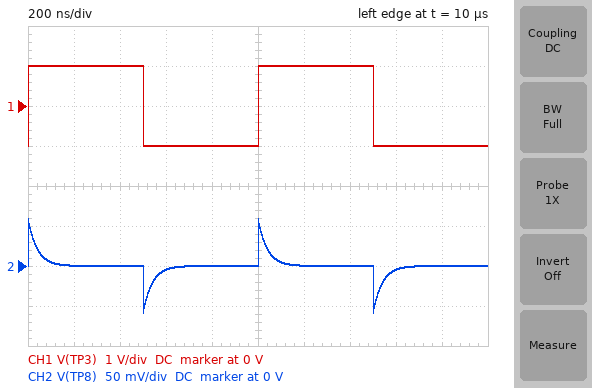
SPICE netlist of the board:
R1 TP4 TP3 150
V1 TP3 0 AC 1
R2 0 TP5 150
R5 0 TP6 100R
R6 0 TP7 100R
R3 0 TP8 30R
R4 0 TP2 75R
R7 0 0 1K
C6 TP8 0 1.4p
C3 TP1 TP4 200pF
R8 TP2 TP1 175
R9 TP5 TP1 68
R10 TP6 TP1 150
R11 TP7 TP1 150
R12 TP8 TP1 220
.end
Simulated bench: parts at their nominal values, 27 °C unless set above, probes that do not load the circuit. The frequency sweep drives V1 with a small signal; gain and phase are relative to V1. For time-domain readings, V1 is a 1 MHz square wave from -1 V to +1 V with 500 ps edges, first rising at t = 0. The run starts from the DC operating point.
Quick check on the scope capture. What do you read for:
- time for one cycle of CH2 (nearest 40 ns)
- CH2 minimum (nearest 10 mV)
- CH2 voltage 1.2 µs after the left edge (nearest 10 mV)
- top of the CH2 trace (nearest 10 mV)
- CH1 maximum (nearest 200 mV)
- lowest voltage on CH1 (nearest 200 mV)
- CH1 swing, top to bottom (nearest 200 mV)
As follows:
1.00 µs
-60 mV
0 V
60 mV
1.0 V
-1.0 V
2.0 V
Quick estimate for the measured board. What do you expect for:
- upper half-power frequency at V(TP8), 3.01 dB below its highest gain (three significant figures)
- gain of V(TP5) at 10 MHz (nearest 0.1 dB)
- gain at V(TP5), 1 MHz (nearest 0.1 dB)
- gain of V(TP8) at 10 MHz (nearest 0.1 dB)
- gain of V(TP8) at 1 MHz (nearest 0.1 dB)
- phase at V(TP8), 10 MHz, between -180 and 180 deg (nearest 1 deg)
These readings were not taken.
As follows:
4.23 GHz
-16.1 dB
-27.8 dB
-31.3 dB
-43.0 dB
22 deg
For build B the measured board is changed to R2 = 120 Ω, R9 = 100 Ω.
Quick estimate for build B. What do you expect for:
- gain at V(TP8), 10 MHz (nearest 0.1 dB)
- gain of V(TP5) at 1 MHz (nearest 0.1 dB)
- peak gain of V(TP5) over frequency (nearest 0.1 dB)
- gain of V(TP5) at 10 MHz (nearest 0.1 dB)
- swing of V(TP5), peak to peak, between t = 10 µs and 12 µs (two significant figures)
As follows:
-31.3 dB
-29.8 dB
-17.5 dB
-18.1 dB
530 mV
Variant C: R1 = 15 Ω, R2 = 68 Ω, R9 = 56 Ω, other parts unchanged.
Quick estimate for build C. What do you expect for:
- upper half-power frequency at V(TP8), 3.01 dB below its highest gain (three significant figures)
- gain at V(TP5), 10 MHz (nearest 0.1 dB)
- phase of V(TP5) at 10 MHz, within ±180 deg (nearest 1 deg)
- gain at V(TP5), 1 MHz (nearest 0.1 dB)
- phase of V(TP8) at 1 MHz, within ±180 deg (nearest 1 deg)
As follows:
4.31 GHz
-12.6 dB
55 deg
-30.9 dB
86 deg
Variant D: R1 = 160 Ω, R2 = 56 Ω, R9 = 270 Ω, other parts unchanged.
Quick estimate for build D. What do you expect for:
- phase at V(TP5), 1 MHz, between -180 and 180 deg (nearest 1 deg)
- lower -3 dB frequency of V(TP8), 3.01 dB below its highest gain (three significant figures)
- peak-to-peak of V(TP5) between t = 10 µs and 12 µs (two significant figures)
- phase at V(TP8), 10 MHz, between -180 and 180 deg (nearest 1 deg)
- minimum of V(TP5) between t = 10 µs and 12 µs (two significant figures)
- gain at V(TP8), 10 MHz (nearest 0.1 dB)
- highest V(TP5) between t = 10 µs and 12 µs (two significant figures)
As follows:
75 deg
3.74 MHz
170 mV
20 deg
-84 mV
-31.1 dB
84 mV
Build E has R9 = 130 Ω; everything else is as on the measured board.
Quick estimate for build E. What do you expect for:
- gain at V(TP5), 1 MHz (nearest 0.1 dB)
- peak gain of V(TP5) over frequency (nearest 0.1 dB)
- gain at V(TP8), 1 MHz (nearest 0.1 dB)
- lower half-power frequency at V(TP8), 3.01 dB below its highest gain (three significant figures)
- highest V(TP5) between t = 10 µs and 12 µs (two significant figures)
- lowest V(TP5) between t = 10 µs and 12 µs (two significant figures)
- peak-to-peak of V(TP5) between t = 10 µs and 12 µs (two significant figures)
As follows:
-29.5 dB
-17.3 dB
-42.5 dB
3.95 MHz
270 mV
-270 mV
540 mV
